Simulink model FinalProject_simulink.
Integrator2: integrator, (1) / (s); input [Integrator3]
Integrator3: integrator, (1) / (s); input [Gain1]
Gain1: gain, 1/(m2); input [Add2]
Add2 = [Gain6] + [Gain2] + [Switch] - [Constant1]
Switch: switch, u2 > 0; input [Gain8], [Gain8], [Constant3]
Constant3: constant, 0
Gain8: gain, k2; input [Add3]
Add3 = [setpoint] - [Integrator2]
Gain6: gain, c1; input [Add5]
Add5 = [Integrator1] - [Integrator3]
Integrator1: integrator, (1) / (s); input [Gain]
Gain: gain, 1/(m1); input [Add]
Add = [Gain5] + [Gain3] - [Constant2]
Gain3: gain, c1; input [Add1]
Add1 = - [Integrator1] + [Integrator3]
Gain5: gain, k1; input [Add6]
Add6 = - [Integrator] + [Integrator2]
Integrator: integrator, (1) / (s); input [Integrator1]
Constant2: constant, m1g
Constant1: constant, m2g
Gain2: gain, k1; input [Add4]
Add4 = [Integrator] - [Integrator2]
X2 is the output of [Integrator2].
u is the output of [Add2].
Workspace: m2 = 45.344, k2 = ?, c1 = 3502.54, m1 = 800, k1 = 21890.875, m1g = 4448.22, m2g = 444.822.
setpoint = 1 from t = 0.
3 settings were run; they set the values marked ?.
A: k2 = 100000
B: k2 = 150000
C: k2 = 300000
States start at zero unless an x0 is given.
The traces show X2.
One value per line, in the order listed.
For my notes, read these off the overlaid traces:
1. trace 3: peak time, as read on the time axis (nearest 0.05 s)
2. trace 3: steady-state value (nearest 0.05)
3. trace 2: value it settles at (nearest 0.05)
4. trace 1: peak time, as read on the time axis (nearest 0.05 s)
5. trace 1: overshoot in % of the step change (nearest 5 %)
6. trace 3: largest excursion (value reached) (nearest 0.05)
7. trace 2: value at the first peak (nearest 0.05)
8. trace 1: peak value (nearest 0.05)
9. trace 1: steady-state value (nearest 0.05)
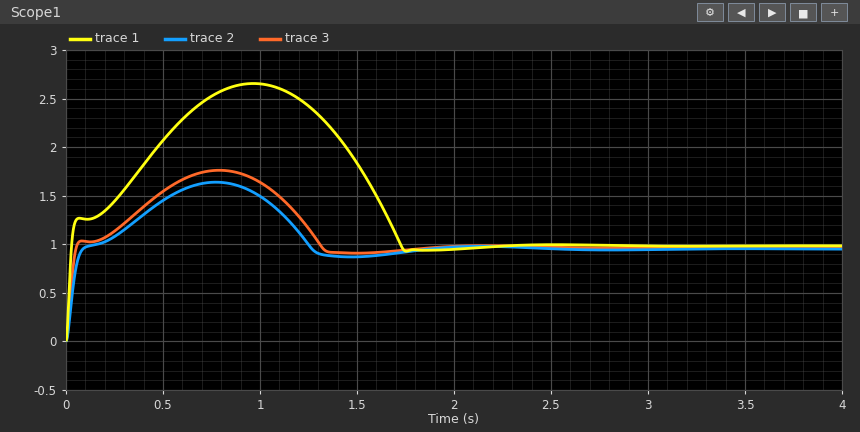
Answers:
0.80 s
0.95
0.95
0.95 s
170 %
1.75
1.65
2.65
1.00
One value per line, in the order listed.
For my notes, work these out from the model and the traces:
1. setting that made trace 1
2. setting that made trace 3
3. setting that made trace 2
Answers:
C
B
A
